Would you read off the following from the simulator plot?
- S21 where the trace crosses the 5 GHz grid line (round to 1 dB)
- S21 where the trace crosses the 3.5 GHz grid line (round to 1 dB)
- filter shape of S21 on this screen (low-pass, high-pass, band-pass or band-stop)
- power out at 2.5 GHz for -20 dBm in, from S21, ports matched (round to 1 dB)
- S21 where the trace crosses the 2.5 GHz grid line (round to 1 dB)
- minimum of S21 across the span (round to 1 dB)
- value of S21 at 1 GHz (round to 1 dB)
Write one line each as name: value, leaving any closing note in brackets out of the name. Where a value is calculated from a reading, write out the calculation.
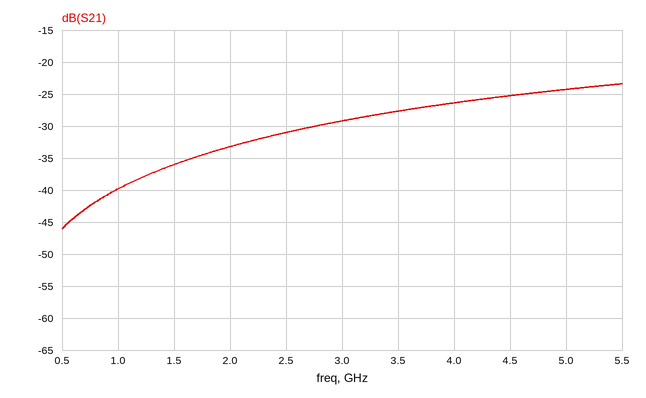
S21 where the trace crosses the 5 GHz grid line: -24 dB
S21 where the trace crosses the 3.5 GHz grid line: -28 dB
filter shape of S21 on this screen: high-pass
power out at 2.5 GHz for -20 dBm in, from S21, ports matched: -20 dBm + (-31 dB) = -51 dBm
S21 where the trace crosses the 2.5 GHz grid line: -31 dB
minimum of S21 across the span: -46 dB
value of S21 at 1 GHz: -40 dB
